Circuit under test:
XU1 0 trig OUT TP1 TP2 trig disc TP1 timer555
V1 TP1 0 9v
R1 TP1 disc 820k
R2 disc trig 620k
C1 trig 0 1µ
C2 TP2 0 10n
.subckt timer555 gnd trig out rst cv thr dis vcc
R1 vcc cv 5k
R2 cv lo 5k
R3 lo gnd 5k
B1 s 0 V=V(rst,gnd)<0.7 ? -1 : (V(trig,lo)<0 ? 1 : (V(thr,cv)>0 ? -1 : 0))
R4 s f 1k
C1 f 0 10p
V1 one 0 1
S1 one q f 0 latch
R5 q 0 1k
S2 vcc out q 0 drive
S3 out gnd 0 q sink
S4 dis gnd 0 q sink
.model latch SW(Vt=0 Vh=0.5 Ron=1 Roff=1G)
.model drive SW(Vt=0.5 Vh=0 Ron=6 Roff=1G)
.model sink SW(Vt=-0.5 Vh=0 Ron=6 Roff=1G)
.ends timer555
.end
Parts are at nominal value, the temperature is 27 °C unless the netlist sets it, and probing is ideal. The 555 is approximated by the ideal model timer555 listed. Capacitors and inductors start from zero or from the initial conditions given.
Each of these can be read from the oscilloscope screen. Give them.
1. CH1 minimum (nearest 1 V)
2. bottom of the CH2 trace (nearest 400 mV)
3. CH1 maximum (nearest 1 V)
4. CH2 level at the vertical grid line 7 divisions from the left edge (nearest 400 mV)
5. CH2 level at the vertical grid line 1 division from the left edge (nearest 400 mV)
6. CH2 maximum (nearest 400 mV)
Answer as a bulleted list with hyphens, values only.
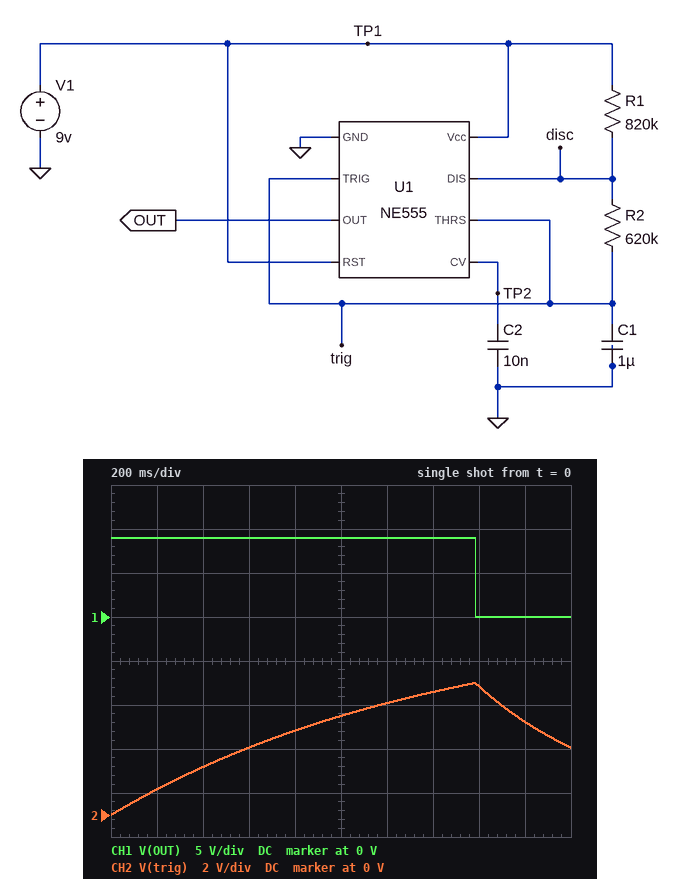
- 0 V
- 0 V
- 9 V
- 5.6 V
- 1.2 V
- 6.0 V
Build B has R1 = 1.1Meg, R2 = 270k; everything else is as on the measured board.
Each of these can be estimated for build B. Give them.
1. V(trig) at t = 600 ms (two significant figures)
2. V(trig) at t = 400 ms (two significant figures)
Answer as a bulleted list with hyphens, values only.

- 3.2 V
- 2.3 V
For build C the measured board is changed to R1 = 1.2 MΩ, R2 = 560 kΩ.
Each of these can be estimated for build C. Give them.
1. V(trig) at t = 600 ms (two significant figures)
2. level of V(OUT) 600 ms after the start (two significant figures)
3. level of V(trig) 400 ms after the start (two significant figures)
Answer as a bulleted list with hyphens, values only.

- 2.6 V
- 9.0 V
- 1.8 V
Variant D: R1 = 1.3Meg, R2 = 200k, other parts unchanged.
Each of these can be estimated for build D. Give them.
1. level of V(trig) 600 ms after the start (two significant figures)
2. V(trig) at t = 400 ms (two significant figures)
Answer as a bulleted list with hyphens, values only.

- 3.0 V
- 2.1 V
